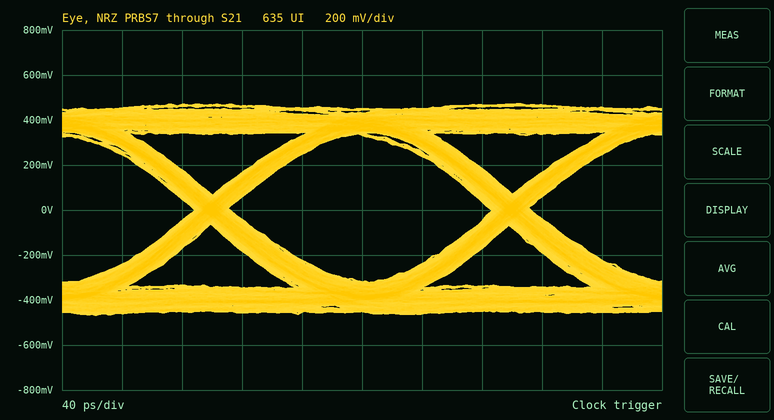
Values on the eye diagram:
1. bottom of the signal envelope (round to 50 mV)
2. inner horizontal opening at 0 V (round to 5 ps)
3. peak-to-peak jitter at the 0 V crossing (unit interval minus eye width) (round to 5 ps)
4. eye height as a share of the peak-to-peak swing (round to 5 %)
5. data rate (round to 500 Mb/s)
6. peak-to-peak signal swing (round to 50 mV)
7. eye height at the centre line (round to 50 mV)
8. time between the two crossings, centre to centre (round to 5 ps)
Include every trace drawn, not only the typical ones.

-450 mV
175 ps
25 ps
70 %
5.0 Gb/s
950 mV
650 mV
200 ps
